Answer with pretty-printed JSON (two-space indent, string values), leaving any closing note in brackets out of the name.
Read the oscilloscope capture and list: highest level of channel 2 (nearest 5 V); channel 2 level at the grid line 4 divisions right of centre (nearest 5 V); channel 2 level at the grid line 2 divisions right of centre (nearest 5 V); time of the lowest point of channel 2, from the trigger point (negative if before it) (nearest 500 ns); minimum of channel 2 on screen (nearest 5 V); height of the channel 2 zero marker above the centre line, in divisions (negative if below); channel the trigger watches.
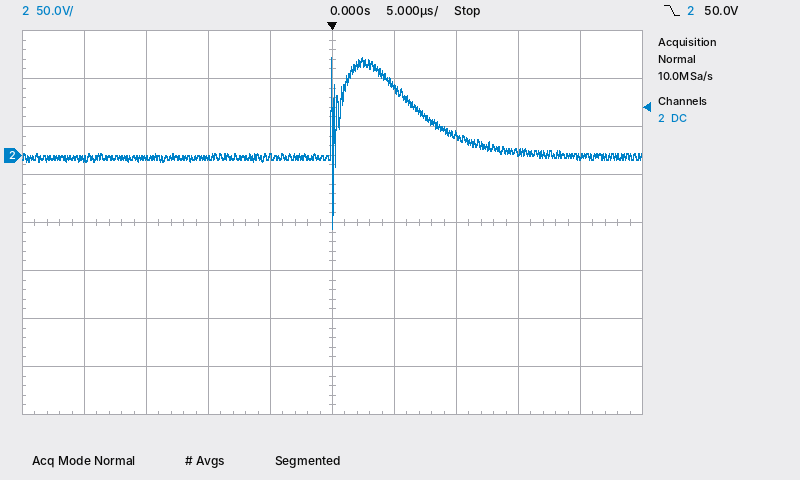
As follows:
{
  "highest level of channel 2": "100 V",
  "channel 2 level at the grid line 4 divisions right of centre": "0 V",
  "channel 2 level at the grid line 2 divisions right of centre": "20 V",
  "time of the lowest point of channel 2, from the trigger point (negative if before it)": "0.0 µs",
  "minimum of channel 2 on screen": "-75 V",
  "height of the channel 2 zero marker above the centre line, in divisions": "+1.4 div",
  "channel the trigger watches": "channel 2"
}
